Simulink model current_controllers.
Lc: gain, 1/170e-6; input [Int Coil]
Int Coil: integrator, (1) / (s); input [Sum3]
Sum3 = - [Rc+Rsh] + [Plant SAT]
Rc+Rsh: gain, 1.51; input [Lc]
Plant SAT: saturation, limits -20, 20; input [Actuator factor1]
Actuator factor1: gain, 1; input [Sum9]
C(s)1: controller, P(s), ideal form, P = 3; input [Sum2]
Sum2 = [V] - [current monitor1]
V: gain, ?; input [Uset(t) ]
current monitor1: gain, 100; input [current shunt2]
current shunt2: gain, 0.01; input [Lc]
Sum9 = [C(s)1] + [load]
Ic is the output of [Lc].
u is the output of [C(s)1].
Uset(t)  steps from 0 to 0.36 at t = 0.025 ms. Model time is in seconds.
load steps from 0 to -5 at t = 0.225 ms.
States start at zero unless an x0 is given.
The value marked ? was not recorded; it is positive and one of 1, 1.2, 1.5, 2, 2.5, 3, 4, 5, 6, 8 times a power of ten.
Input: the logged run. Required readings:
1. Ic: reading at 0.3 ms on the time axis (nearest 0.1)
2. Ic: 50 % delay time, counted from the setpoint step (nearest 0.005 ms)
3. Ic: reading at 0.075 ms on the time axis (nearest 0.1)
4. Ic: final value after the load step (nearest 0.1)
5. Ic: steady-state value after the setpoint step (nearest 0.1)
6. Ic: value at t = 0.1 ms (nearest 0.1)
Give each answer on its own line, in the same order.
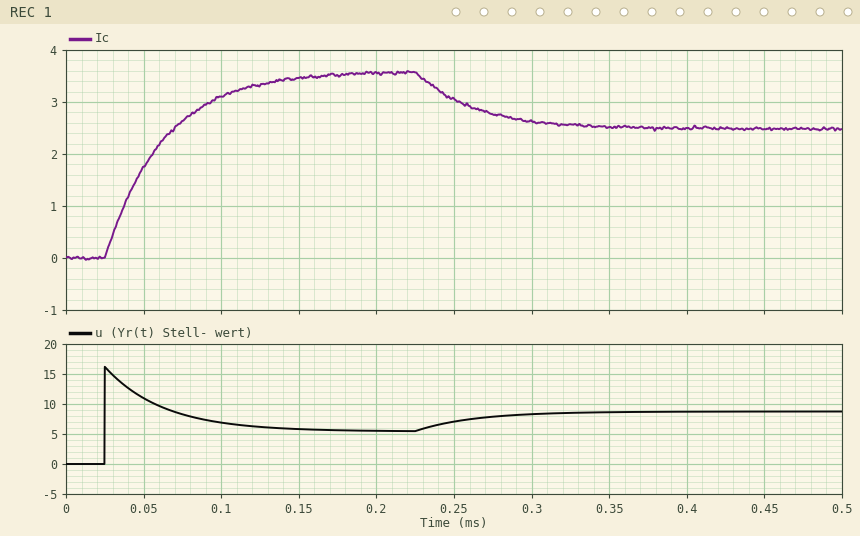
2.6
0.025 ms
2.6
2.5
3.6
3.1
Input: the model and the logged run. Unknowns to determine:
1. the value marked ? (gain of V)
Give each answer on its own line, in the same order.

15
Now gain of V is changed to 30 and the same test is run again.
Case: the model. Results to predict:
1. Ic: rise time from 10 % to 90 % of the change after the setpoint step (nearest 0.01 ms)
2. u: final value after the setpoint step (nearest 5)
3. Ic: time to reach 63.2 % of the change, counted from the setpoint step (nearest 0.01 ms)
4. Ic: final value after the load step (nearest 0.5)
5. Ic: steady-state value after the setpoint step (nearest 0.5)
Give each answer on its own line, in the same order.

0.09 ms
10
0.05 ms
6.0
7.0
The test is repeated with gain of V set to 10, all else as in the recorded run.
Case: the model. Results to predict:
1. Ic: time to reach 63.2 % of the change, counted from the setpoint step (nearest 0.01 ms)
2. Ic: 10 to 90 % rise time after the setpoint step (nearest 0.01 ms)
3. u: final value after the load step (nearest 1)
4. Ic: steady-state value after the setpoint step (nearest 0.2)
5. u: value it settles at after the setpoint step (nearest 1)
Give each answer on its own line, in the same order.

0.04 ms
0.08 ms
7
2.4
4
